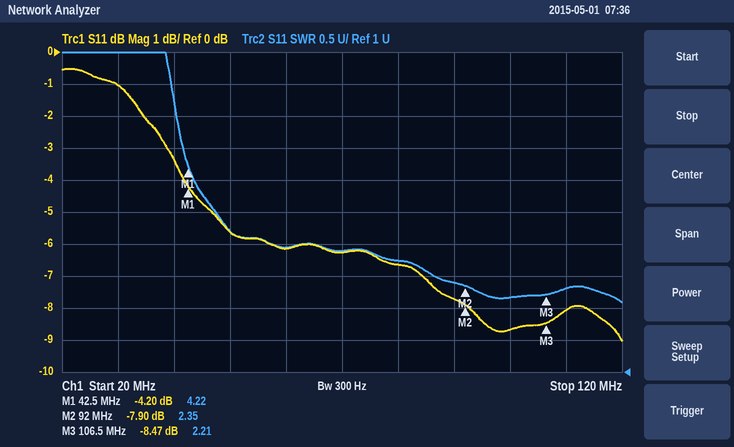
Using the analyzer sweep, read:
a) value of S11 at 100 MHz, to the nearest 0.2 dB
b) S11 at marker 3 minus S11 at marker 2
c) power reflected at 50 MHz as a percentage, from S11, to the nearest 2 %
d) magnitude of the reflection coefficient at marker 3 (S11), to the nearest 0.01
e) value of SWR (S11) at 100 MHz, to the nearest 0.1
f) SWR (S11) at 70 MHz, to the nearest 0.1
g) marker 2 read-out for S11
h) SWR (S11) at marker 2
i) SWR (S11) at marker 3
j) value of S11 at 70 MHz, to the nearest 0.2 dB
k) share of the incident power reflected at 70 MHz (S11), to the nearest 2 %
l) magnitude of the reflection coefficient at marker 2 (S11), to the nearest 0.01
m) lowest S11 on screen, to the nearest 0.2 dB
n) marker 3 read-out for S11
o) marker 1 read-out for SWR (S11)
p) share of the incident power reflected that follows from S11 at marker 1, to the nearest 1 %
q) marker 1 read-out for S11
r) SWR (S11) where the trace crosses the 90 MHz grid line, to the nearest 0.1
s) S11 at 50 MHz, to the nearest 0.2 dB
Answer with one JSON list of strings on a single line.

["-8.6 dB", "-0.57 dB", "28 %", "0.38", "2.2", "2.9", "-7.90 dB", "2.35", "2.21", "-6.2 dB", "24 %", "0.40", "-9.0 dB", "-8.47 dB", "4.22", "38 %", "-4.20 dB", "2.4", "-5.6 dB"]
